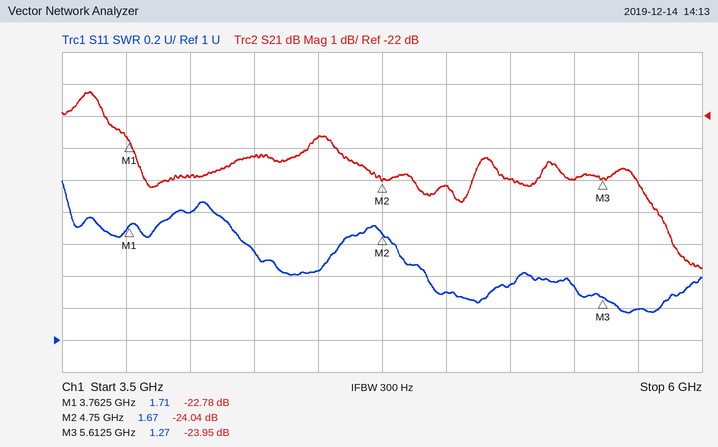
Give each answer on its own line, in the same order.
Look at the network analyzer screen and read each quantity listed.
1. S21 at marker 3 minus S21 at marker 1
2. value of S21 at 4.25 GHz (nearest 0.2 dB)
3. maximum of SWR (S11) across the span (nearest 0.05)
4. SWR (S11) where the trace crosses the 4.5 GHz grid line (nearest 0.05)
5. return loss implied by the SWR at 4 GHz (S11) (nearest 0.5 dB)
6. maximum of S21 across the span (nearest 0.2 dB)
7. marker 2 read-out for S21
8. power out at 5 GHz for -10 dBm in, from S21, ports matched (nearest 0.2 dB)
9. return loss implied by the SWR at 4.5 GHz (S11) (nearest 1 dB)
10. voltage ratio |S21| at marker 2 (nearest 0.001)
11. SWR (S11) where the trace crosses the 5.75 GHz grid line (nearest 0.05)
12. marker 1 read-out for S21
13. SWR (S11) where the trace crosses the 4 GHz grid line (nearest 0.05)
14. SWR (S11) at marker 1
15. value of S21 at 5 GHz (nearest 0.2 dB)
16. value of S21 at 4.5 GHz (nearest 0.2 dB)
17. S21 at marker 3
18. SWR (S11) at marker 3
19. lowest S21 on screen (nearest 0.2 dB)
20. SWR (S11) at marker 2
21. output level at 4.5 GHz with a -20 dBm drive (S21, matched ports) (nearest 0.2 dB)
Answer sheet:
-1.17 dB
-23.2 dB
2.00
1.45
11.0 dB
-21.2 dB
-24.04 dB
-34.2 dBm
15 dB
0.063
1.20
-22.78 dB
1.80
1.71
-24.2 dB
-22.6 dB
-23.95 dB
1.27
-26.8 dB
1.67
-42.6 dBm
